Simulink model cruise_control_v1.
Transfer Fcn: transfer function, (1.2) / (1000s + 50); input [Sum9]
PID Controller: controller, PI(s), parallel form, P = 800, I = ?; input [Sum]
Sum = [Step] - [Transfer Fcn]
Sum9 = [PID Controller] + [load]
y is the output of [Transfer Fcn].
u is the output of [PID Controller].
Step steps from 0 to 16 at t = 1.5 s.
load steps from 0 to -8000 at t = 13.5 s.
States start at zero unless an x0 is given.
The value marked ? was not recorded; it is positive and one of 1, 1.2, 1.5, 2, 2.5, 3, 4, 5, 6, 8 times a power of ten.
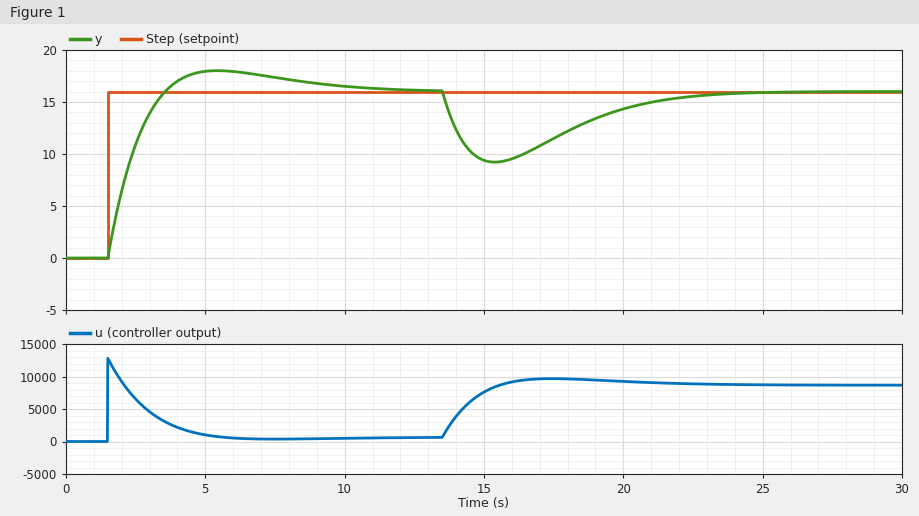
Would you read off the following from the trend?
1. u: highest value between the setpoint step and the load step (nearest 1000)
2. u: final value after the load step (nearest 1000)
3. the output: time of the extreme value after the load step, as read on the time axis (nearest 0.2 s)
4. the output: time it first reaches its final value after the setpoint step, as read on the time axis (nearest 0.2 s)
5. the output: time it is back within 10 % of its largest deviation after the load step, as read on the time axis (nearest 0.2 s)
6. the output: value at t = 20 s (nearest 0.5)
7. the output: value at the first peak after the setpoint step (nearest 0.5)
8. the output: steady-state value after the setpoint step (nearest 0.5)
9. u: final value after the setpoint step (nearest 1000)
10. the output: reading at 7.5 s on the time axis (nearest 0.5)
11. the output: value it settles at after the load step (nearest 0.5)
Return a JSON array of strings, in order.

["13000", "9000", "15.4 s", "3.6 s", "21.8 s", "14.5", "18.0", "16.0", "1000", "17.5", "16.0"]
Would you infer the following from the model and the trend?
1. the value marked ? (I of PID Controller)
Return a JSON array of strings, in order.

["250"]
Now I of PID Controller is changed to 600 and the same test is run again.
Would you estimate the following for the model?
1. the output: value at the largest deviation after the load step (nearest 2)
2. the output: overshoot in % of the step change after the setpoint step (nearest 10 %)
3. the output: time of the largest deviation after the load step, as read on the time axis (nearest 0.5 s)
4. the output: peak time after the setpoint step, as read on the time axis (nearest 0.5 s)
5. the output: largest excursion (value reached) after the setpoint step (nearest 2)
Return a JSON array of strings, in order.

["10", "20 %", "15.0 s", "4.5 s", "20"]
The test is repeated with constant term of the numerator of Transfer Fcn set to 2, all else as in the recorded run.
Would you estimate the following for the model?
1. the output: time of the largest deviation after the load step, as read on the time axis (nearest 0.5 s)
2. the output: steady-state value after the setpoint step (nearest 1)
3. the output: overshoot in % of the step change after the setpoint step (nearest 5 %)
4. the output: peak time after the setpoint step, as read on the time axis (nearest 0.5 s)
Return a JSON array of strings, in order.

["15.0 s", "16", "10 %", "4.5 s"]
